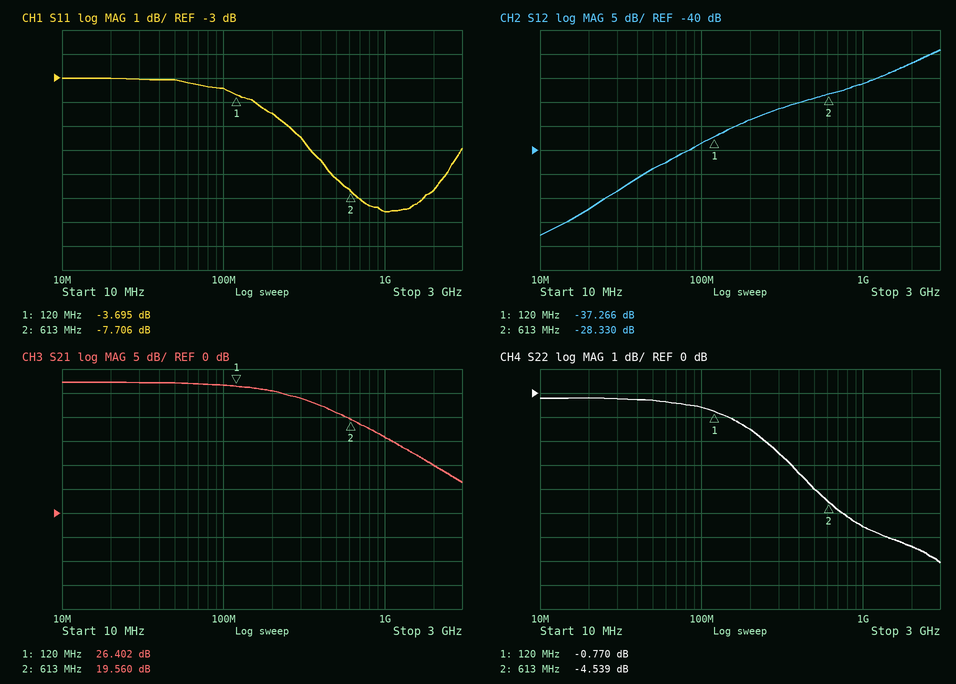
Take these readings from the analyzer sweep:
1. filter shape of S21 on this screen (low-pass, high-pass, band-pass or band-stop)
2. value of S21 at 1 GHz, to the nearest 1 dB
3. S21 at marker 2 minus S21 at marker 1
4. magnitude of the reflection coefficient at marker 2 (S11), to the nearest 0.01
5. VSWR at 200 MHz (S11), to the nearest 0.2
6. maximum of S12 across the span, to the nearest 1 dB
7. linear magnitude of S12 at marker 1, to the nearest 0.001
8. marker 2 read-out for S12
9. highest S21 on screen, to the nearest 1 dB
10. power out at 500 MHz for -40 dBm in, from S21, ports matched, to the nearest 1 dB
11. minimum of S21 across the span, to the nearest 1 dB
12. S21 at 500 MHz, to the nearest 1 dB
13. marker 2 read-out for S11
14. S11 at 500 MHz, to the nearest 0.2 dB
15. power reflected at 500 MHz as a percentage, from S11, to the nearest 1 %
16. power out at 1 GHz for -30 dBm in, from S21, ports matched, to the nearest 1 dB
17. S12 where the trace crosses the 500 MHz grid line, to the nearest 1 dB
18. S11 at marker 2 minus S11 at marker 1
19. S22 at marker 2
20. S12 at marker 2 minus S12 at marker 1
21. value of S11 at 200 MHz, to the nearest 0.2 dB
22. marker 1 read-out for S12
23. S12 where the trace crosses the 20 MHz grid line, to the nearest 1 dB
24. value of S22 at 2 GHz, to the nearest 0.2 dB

low-pass
16 dB
-6.842 dB
0.41
4.0
-19 dB
0.014
-28.330 dB
27 dB
-19 dBm
6 dB
21 dB
-7.706 dB
-7.2 dB
19 %
-14 dBm
-29 dB
-4.011 dB
-4.539 dB
8.936 dB
-4.4 dB
-37.266 dB
-52 dB
-6.4 dB
